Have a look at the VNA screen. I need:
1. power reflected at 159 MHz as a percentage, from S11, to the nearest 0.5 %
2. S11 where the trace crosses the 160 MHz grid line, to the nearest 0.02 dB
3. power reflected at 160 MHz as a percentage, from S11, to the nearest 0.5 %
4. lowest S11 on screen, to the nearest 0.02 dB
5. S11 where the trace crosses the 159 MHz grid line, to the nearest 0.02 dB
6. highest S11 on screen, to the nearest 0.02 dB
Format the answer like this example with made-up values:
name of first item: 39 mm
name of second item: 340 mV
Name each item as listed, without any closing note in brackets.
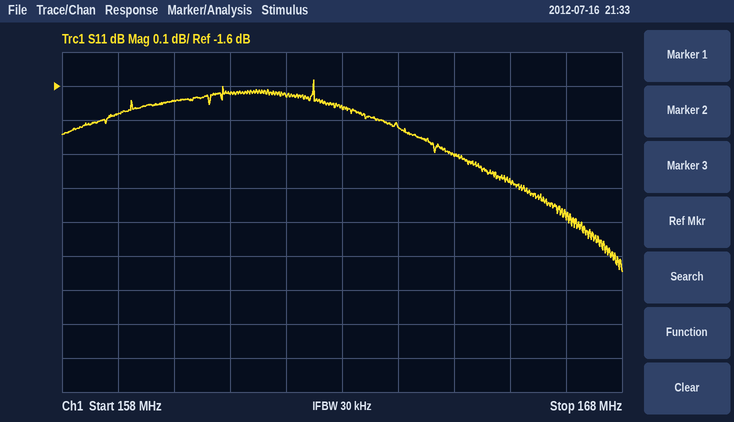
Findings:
power reflected at 159 MHz as a percentage, from S11, to the nearest 0.5 %: 68.0 %
S11 where the trace crosses the 160 MHz grid line, to the nearest 0.02 dB: -1.64 dB
power reflected at 160 MHz as a percentage, from S11, to the nearest 0.5 %: 68.5 %
lowest S11 on screen, to the nearest 0.02 dB: -2.14 dB
S11 where the trace crosses the 159 MHz grid line, to the nearest 0.02 dB: -1.68 dB
highest S11 on screen, to the nearest 0.02 dB: -1.58 dB
